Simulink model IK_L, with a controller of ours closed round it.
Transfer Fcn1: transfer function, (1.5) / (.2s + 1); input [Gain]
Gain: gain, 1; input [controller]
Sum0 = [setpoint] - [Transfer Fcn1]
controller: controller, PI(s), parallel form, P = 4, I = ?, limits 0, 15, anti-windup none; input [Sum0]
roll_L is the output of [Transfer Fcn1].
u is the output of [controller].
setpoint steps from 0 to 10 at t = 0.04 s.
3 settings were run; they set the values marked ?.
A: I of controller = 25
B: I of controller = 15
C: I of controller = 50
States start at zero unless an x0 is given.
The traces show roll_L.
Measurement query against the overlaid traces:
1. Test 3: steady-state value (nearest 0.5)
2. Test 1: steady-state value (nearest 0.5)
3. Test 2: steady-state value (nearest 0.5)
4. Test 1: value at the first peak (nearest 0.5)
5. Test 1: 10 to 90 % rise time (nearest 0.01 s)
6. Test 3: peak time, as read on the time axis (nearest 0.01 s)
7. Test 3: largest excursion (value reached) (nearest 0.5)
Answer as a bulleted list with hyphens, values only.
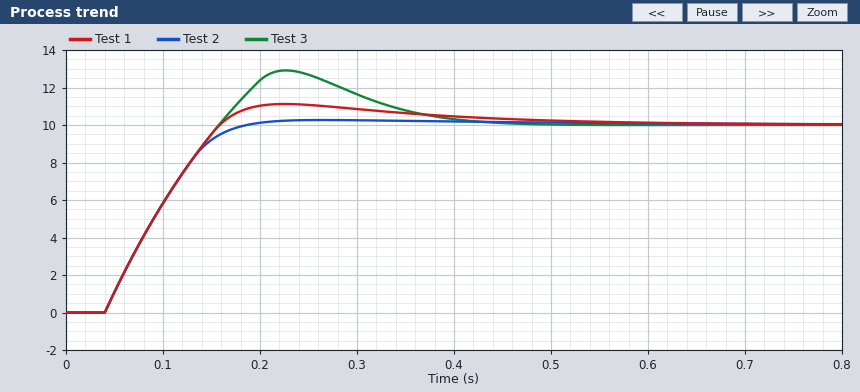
- 10.0
- 10.0
- 10.0
- 11.0
- 0.09 s
- 0.23 s
- 13.0
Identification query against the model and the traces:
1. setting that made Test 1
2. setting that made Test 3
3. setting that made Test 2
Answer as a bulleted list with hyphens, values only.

- A
- C
- B
